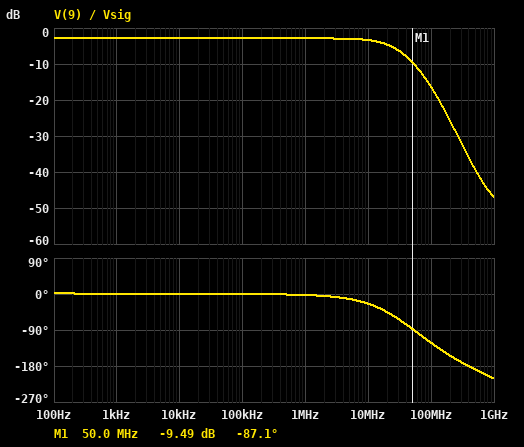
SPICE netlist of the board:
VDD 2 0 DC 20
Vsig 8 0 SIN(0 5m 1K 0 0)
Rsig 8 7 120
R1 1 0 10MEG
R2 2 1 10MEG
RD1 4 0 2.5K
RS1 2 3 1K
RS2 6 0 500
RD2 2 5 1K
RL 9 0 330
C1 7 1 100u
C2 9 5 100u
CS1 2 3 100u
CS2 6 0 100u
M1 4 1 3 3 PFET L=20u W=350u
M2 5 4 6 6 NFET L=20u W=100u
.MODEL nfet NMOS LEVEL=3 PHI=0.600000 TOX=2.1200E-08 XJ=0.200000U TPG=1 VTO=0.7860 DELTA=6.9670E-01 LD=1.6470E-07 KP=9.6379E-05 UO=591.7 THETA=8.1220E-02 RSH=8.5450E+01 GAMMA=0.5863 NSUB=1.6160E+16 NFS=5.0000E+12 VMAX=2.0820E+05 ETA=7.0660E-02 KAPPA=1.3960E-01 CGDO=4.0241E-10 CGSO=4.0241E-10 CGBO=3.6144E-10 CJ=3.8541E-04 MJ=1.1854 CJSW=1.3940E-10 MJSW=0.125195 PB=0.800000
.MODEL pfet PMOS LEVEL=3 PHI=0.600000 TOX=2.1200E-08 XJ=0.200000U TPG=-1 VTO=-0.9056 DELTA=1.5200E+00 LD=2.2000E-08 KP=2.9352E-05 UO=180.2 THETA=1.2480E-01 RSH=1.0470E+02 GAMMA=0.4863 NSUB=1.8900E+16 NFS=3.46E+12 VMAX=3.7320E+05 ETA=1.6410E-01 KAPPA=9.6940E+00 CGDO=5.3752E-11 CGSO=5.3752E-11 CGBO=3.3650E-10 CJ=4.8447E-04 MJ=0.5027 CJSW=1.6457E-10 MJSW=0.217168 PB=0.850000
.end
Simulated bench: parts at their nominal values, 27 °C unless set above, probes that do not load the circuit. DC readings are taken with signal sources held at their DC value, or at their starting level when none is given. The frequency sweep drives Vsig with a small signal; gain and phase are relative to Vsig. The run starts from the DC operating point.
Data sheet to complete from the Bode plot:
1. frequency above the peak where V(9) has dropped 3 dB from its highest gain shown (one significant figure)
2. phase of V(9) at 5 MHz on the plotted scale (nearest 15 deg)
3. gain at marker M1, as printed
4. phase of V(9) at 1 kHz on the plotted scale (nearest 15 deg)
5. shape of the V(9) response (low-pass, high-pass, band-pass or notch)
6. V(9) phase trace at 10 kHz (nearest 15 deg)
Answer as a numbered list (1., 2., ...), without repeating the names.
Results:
1. 30 MHz
2. -15 deg
3. -9.49 dB
4. 0 deg
5. low-pass
6. 0 deg
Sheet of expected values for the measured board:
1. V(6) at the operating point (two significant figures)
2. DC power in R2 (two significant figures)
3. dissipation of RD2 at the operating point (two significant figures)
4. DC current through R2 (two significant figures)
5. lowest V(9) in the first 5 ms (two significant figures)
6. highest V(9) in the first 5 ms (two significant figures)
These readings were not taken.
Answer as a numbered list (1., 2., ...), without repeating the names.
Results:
1. 2.1 V
2. 10 µW
3. 18 mW
4. 1.0 µA
5. -3.6 mV
6. 3.6 mV
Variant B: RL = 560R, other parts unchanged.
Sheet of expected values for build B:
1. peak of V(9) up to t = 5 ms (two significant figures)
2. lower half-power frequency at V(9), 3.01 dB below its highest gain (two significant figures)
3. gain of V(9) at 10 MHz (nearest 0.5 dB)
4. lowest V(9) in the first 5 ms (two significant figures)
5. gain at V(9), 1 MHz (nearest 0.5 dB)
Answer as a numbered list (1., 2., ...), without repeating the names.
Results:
1. 5.2 mV
2. 4.7 Hz
3. 0 dB
4. -5.2 mV
5. 0.5 dB
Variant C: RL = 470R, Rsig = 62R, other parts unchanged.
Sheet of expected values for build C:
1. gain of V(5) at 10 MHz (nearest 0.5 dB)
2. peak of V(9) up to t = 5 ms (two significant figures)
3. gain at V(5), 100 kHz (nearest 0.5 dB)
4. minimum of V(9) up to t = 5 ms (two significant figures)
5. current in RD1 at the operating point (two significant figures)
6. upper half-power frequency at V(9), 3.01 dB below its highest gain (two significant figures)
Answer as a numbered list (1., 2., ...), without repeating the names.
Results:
1. -1.0 dB
2. 4.6 mV
3. -0.5 dB
4. -4.7 mV
5. 3.6 mA
6. 29 MHz
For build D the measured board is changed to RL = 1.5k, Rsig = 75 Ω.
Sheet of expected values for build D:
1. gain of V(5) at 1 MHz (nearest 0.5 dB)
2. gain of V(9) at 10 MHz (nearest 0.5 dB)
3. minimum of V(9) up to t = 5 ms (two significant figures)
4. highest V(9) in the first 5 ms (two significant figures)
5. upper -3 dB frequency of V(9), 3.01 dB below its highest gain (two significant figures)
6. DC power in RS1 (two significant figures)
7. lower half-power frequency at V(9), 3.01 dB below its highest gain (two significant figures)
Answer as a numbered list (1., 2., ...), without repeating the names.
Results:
1. 5.0 dB
2. 4.5 dB
3. -8.7 mV
4. 8.7 mV
5. 29 MHz
6. 13 mW
7. 4.6 Hz
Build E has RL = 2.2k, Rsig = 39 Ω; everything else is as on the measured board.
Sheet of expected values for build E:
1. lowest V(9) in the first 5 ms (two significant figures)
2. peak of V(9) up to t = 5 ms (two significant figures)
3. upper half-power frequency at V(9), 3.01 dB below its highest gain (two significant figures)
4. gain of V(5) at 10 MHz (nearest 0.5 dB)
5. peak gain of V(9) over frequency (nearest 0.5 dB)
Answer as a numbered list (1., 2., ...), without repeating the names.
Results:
1. -10 mV
2. 9.9 mV
3. 29 MHz
4. 5.5 dB
5. 6.0 dB
